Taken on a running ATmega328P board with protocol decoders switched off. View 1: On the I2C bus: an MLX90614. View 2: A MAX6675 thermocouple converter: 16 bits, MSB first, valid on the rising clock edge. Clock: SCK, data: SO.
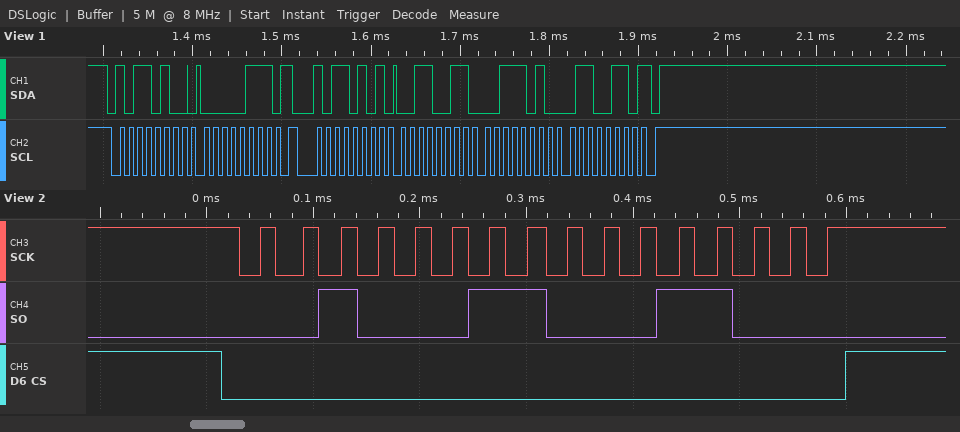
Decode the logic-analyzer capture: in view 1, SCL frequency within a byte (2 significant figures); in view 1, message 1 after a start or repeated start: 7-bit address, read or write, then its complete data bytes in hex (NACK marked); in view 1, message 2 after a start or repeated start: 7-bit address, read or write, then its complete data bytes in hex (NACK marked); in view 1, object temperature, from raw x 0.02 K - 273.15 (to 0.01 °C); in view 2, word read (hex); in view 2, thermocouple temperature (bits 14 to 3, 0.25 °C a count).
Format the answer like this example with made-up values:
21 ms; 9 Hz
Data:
100 kHz; 0x5A write: 07; 0x5A read: 33 3A 66 NACK; 24.83 °C; 0x2318; 280.75 °C
